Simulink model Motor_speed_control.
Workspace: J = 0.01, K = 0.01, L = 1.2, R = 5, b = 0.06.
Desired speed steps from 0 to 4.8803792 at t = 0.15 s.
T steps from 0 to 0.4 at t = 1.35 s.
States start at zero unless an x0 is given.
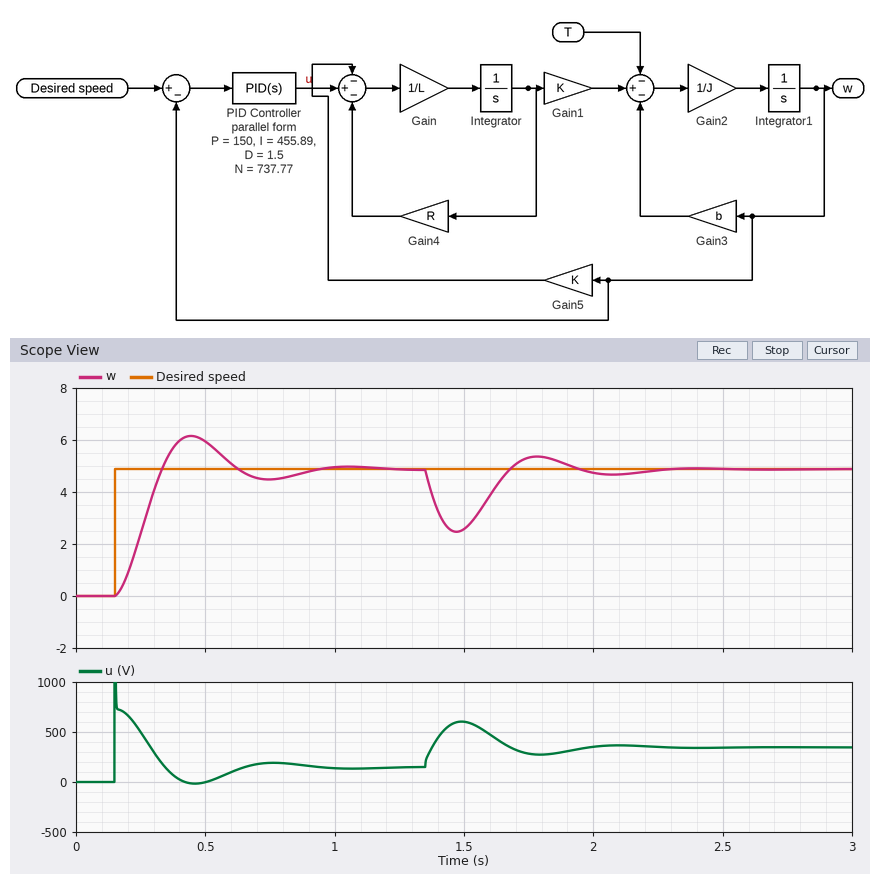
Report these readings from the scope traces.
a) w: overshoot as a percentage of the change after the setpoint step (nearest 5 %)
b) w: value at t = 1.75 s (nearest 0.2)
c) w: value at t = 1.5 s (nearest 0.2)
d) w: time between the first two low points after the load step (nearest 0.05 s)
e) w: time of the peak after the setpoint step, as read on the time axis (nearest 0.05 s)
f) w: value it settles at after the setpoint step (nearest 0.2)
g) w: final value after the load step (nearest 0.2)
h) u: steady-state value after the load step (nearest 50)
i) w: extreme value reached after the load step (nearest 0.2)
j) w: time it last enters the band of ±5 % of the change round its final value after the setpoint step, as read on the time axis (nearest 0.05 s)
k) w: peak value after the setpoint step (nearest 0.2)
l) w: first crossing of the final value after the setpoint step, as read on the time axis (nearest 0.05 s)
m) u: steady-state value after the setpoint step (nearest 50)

25 %
5.4
2.6
0.60 s
0.45 s
4.8
4.8
350
2.4
0.85 s
6.2
0.35 s
150
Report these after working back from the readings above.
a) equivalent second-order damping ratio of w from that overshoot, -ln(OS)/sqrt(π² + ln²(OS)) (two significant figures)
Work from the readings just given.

0.40
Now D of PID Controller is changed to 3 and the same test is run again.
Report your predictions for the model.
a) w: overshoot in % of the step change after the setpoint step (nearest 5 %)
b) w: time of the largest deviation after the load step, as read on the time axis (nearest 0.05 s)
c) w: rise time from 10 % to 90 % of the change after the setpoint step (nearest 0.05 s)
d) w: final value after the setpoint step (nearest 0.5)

20 %
1.45 s
0.15 s
5.0
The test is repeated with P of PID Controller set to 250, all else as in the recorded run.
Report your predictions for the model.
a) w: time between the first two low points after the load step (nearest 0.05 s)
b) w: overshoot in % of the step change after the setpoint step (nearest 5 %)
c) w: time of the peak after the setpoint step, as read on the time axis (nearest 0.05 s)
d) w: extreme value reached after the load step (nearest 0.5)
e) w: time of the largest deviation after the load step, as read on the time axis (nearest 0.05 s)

0.45 s
30 %
0.35 s
3.0
1.45 s
